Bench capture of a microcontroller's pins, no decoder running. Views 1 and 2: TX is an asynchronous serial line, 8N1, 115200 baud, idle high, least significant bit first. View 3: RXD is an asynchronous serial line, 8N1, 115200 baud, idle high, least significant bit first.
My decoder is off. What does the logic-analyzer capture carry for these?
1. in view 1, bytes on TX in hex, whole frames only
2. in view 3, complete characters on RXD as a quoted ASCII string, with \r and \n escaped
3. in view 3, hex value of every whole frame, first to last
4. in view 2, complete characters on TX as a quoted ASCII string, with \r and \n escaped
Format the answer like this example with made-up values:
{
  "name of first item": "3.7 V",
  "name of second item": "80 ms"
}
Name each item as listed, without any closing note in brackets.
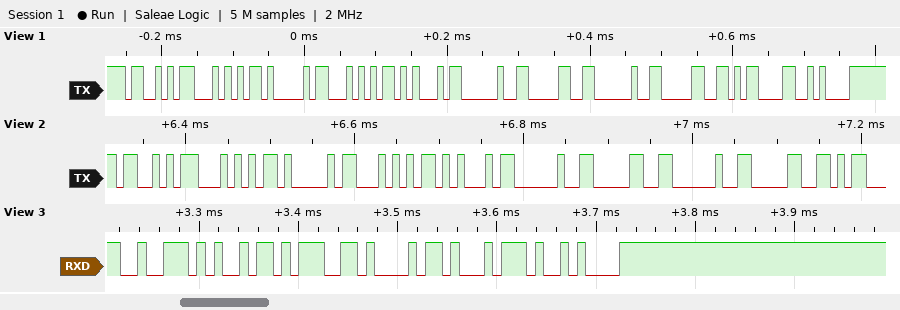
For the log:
{
  "in view 1, bytes on TX in hex, whole frames only": "0x53 0x54 0x41 0x54 0x45 0x20 0x30 0x20 0x30 0x0D 0x0A",
  "in view 3, complete characters on RXD as a quoted ASCII string, with \\r and \\n escaped": "\"right\\n\"",
  "in view 3, hex value of every whole frame, first to last": "72 69 67 68 74 0A",
  "in view 2, complete characters on TX as a quoted ASCII string, with \\r and \\n escaped": "\"STATE 0 0\""
}
